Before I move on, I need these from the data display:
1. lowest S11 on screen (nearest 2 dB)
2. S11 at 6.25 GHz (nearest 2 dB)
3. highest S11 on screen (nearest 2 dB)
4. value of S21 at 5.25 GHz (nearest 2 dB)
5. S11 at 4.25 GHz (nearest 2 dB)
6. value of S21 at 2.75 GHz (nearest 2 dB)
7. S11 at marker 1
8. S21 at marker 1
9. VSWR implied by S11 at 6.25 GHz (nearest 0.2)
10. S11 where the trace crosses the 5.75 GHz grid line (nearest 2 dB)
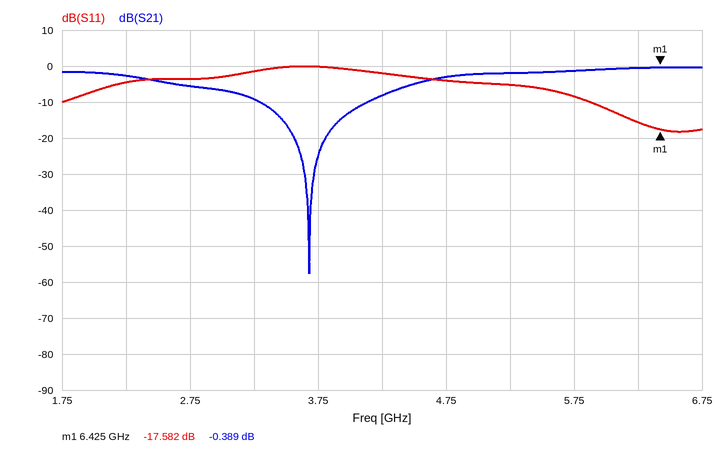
-18 dB
-16 dB
0 dB
-2 dB
-2 dB
-6 dB
-17.582 dB
-0.389 dB
1.4
-8 dB
